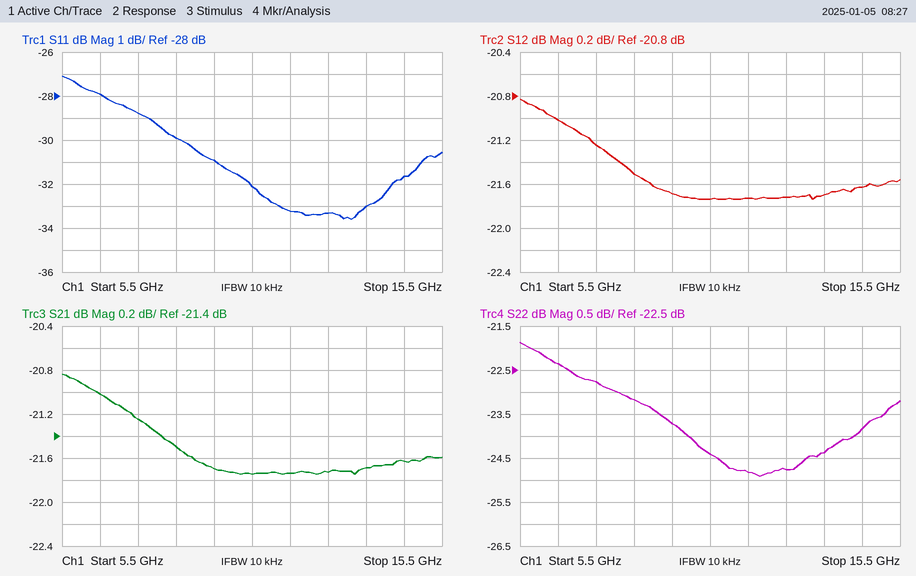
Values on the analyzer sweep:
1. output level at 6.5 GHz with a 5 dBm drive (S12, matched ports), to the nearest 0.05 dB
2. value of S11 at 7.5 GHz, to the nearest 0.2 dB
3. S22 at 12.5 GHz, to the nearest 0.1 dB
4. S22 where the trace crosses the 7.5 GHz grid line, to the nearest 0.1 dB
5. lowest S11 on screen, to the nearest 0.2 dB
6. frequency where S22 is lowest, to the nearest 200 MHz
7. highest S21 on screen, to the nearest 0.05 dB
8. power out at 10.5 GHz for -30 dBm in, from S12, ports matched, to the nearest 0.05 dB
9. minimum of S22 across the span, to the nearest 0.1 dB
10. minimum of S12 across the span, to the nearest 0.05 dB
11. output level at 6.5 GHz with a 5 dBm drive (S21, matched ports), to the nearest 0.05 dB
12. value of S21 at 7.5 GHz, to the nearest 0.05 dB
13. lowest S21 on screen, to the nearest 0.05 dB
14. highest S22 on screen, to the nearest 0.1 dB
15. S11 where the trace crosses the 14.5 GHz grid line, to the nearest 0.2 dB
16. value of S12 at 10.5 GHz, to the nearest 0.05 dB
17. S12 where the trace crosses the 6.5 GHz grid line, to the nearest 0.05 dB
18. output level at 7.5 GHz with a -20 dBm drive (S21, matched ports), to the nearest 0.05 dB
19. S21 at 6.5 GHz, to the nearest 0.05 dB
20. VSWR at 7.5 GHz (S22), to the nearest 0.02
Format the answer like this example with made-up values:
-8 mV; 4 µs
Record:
-16.00 dBm; -28.8 dB; -24.8 dB; -22.8 dB; -33.6 dB; 11.8 GHz; -20.85 dB; -51.75 dBm; -24.9 dB; -21.75 dB; -16.00 dBm; -21.25 dB; -21.75 dB; -21.9 dB; -31.6 dB; -21.75 dB; -21.00 dB; -41.25 dBm; -21.00 dB; 1.16
